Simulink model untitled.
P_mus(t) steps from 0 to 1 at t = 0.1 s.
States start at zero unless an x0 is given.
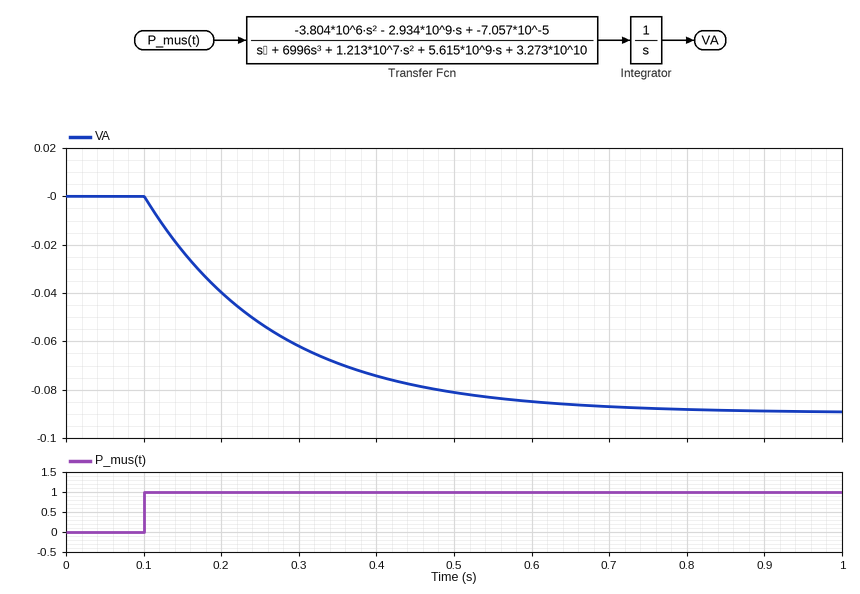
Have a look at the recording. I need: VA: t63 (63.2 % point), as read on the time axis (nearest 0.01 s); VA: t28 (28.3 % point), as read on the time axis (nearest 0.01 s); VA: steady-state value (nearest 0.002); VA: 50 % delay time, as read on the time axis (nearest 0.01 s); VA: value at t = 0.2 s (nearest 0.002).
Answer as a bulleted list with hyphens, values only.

- 0.27 s
- 0.16 s
- -0.090
- 0.22 s
- -0.040
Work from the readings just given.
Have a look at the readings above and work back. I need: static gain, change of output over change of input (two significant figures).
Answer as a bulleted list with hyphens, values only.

- -0.090
